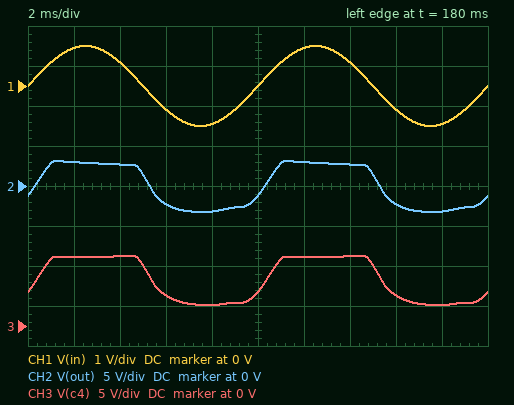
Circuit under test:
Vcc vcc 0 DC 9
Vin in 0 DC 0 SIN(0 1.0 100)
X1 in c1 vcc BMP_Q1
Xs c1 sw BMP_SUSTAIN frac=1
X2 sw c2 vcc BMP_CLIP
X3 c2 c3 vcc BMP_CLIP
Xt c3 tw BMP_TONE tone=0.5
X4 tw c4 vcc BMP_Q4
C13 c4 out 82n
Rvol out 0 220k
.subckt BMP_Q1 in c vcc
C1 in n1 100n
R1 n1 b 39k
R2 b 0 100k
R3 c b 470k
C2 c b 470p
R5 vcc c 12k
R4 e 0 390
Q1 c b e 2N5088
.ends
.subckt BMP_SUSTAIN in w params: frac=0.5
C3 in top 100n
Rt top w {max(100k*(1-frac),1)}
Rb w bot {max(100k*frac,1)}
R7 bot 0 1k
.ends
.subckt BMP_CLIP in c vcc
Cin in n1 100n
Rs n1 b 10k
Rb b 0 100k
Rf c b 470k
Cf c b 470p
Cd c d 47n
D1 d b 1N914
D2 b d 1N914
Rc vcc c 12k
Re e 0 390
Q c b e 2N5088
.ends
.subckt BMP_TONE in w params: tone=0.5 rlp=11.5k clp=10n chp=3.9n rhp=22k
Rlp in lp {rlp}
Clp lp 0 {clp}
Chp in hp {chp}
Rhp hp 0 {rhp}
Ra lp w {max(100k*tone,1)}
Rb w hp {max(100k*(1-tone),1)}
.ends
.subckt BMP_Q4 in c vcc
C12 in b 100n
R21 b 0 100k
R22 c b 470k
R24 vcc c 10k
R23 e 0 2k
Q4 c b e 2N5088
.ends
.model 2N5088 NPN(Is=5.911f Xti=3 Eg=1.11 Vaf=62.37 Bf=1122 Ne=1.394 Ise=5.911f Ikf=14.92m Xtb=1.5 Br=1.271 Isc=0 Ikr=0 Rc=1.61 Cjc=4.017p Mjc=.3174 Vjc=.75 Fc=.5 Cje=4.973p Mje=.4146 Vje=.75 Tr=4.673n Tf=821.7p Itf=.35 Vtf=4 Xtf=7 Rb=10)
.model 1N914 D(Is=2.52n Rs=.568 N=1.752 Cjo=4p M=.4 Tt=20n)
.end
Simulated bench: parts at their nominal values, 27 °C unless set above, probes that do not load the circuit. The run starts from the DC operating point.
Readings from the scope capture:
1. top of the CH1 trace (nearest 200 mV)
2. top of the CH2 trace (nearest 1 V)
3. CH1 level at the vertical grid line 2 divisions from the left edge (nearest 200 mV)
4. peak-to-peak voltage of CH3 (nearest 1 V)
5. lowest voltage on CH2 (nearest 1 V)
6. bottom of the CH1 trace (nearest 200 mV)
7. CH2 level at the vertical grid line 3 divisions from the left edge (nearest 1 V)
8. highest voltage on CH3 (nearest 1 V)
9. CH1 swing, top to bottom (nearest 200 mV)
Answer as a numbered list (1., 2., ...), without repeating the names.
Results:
1. 1.0 V
2. 3 V
3. 600 mV
4. 6 V
5. -3 V
6. -1.0 V
7. -2 V
8. 9 V
9. 2.0 V
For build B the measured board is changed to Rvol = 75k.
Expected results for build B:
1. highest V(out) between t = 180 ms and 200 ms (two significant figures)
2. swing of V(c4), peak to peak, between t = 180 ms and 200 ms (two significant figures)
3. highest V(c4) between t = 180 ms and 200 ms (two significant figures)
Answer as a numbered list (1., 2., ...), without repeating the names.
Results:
1. 3.2 V
2. 5.8 V
3. 8.6 V
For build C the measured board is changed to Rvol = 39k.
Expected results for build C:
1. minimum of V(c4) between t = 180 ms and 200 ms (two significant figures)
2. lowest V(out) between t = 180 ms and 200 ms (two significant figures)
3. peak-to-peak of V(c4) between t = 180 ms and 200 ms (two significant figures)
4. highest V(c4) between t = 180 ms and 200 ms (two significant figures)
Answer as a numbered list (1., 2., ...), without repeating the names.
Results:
1. 2.9 V
2. -2.8 V
3. 5.6 V
4. 8.5 V
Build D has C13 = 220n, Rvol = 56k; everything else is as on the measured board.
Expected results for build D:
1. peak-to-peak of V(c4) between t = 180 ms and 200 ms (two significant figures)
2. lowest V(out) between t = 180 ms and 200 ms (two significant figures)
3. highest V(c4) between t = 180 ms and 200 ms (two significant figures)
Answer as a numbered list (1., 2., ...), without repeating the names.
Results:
1. 5.6 V
2. -2.9 V
3. 8.4 V
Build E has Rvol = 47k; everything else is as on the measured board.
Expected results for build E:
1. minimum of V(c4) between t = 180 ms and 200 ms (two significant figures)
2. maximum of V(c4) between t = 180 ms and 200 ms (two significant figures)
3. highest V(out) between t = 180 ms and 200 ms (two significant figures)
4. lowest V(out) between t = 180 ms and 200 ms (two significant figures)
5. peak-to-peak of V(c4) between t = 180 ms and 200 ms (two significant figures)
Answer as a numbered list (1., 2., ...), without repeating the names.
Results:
1. 2.9 V
2. 8.5 V
3. 3.2 V
4. -2.9 V
5. 5.6 V
